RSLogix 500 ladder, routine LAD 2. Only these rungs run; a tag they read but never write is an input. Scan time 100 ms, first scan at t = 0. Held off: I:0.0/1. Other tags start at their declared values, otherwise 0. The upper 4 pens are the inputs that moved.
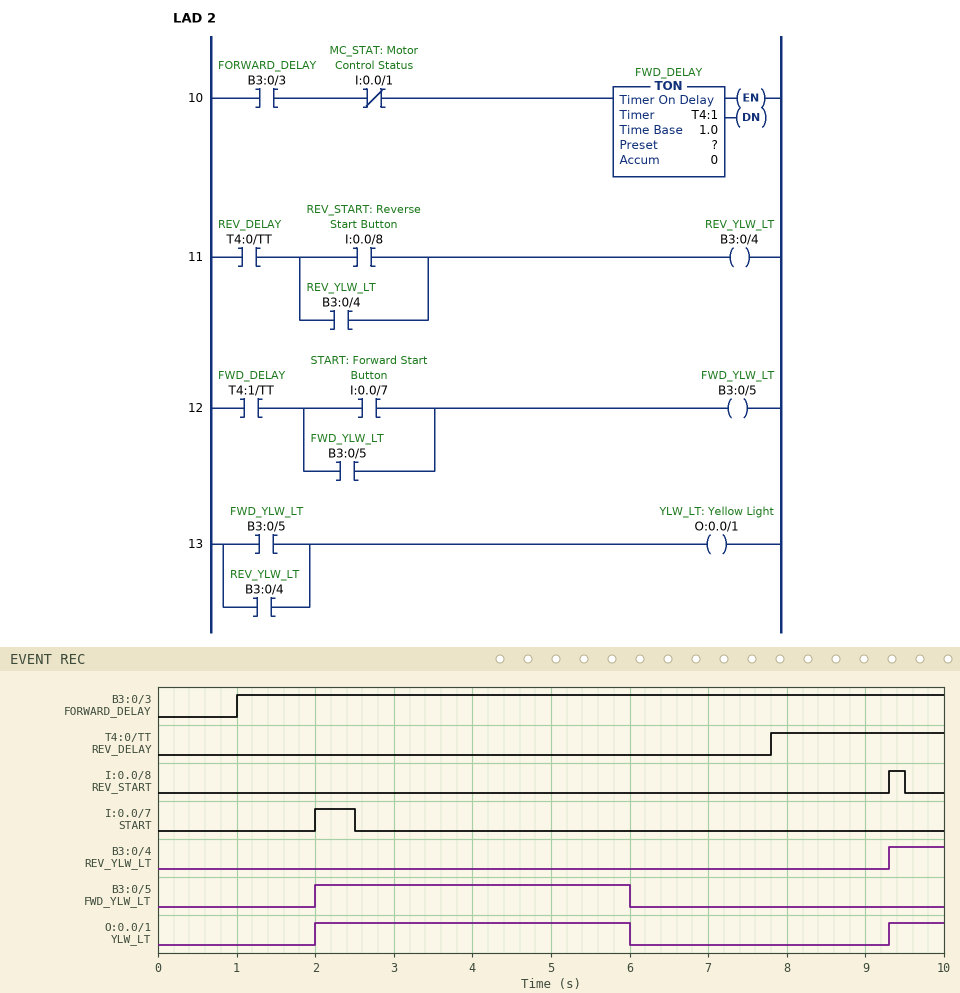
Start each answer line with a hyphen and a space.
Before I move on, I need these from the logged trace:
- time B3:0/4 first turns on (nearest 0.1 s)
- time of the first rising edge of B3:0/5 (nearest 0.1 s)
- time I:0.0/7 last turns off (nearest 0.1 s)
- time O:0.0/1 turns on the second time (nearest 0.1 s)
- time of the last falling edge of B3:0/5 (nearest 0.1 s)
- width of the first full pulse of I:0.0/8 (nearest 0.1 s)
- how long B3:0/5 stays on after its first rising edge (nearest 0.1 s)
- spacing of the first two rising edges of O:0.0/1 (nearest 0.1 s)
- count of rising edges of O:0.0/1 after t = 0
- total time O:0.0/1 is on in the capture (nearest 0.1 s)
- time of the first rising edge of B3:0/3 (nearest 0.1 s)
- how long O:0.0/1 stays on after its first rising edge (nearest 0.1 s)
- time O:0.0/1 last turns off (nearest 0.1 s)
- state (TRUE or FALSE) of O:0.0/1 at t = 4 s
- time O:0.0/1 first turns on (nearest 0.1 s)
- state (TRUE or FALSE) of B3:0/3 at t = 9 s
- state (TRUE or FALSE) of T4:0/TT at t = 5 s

- 9.3 s
- 2.0 s
- 2.5 s
- 9.3 s
- 6.0 s
- 0.2 s
- 4.0 s
- 7.3 s
- 2
- 4.7 s
- 1.0 s
- 4.0 s
- 6.0 s
- TRUE
- 2.0 s
- TRUE
- FALSE
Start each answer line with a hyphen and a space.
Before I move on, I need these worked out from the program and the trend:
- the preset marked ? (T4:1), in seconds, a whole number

- 5 s
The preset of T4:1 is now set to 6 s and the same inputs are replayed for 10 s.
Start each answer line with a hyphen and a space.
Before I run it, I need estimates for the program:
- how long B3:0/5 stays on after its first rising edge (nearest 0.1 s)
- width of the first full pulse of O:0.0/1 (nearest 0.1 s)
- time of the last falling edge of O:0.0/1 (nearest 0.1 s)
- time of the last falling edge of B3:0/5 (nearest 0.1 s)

- 5.0 s
- 5.0 s
- 7.0 s
- 7.0 s
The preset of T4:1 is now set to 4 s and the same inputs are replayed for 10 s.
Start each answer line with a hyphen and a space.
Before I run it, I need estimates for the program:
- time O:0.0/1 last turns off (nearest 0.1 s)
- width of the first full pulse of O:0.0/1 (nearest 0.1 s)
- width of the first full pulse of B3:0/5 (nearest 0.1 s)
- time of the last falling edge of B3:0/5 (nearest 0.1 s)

- 5.0 s
- 3.0 s
- 3.0 s
- 5.0 s
